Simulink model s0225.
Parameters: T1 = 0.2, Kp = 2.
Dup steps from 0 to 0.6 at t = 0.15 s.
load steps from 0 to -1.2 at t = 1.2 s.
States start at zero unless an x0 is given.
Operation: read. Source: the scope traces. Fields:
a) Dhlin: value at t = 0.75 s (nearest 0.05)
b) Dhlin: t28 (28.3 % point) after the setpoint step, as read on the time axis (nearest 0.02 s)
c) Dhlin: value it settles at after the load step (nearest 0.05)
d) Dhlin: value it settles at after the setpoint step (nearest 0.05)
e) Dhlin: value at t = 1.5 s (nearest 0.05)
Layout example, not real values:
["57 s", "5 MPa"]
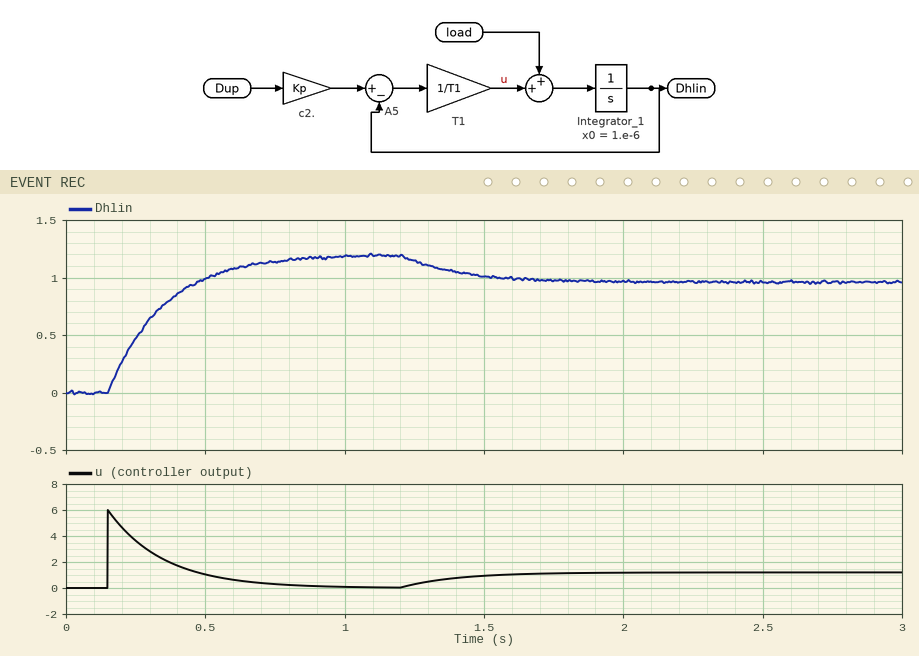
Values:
["1.15", "0.22 s", "0.95", "1.20", "1.00"]
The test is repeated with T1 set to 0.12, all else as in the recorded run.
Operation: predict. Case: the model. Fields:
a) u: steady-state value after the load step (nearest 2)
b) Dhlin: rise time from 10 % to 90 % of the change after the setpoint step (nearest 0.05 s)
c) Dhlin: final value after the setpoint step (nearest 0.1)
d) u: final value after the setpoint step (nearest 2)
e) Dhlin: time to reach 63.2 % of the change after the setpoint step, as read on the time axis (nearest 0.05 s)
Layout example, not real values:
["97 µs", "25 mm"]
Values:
["2", "0.25 s", "1.2", "0", "0.25 s"]
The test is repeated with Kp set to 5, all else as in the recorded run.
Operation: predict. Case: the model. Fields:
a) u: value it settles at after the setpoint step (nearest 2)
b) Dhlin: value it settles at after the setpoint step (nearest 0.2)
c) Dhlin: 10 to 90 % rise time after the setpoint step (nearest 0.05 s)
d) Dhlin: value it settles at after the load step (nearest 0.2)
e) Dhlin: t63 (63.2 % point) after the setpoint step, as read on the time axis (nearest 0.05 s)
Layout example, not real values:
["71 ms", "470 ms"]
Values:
["0", "3.0", "0.45 s", "2.8", "0.35 s"]
